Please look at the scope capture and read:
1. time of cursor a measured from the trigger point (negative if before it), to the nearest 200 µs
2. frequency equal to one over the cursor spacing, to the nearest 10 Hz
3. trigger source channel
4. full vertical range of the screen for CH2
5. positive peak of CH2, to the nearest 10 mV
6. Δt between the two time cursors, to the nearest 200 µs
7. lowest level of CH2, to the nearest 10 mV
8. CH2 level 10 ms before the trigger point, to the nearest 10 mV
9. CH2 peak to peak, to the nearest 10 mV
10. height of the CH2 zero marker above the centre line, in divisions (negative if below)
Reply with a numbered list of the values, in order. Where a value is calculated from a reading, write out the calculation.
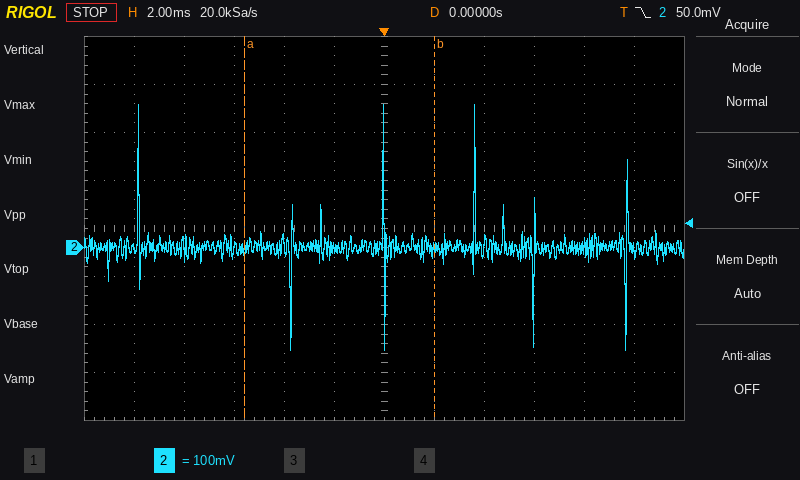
1. -5.6 ms
2. 1 / 7.6 ms ≈ 130 Hz
3. CH2
4. 800 mV
5. 300 mV
6. 7.6 ms
7. -210 mV
8. 0 mV
9. 300 mV − (-210 mV) = 510 mV
10. -0.4 div
